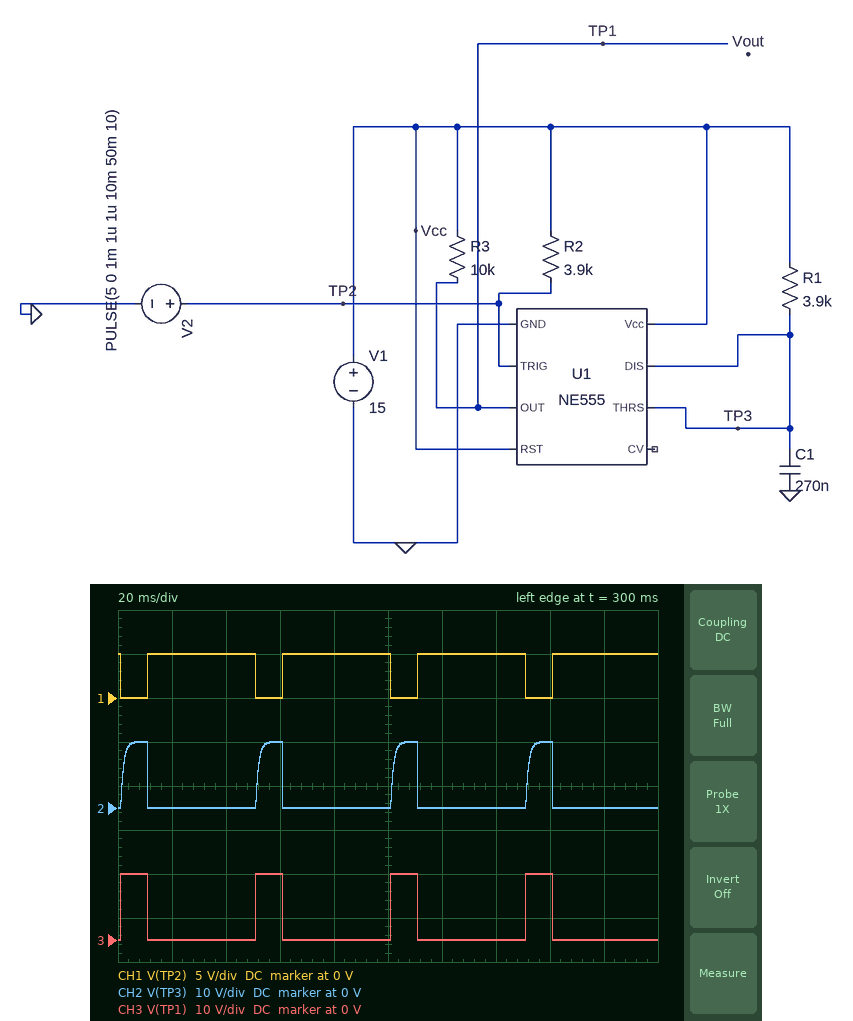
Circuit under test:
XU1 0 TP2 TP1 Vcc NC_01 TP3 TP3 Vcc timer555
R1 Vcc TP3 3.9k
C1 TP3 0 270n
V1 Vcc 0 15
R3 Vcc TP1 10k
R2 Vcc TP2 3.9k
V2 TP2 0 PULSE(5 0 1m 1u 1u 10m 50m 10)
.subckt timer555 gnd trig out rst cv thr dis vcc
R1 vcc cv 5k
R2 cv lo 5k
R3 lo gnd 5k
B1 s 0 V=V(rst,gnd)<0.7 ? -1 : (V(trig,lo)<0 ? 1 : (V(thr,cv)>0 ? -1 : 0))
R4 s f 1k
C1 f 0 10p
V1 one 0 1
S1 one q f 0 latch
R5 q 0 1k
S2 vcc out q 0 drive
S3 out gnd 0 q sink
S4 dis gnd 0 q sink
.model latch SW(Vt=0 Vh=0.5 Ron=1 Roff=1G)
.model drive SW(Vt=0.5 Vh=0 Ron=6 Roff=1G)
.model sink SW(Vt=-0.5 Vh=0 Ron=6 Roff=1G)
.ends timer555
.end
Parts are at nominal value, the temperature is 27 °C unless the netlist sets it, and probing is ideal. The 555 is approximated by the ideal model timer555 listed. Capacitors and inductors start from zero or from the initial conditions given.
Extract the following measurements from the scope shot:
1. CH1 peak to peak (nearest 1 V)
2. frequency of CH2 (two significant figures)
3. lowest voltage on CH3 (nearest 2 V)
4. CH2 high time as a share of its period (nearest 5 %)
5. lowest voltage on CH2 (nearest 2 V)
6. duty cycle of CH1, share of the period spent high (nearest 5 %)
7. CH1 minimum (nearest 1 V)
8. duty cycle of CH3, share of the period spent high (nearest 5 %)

5 V
20 Hz
0 V
20 %
0 V
80 %
0 V
20 %
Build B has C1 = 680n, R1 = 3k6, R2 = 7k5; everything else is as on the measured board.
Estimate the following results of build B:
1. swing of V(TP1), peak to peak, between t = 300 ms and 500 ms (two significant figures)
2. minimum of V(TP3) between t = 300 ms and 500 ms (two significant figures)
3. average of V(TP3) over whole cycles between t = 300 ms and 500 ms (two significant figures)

15 V
25 mV
2.3 V
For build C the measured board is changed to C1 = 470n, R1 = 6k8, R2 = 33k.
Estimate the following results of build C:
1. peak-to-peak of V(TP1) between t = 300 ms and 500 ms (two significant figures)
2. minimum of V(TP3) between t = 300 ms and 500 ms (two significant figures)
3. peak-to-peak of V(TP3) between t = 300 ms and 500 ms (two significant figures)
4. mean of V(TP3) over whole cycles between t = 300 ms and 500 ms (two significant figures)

15 V
13 mV
14 V
2.1 V
